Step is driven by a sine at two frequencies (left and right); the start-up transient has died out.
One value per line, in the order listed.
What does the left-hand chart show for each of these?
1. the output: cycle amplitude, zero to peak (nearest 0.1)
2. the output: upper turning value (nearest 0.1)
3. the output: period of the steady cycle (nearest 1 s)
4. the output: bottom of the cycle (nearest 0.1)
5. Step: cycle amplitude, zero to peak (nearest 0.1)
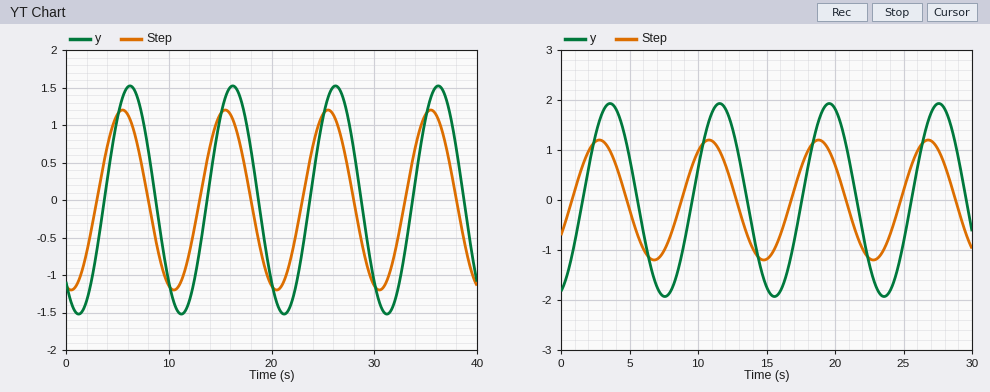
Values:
1.5
1.5
10 s
-1.5
1.2
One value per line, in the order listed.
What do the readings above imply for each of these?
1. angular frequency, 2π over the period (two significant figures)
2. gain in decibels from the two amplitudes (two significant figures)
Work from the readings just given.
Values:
0.63 rad/s
1.9 dB
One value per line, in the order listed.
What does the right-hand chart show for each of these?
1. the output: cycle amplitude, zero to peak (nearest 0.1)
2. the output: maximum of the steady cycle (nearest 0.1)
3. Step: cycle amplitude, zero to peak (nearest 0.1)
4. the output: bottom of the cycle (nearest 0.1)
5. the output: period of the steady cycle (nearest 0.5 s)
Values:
1.9
1.9
1.2
-1.9
8.0 s
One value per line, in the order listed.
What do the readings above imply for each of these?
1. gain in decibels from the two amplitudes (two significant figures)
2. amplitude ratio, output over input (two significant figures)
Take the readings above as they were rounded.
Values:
4.0 dB
1.6
